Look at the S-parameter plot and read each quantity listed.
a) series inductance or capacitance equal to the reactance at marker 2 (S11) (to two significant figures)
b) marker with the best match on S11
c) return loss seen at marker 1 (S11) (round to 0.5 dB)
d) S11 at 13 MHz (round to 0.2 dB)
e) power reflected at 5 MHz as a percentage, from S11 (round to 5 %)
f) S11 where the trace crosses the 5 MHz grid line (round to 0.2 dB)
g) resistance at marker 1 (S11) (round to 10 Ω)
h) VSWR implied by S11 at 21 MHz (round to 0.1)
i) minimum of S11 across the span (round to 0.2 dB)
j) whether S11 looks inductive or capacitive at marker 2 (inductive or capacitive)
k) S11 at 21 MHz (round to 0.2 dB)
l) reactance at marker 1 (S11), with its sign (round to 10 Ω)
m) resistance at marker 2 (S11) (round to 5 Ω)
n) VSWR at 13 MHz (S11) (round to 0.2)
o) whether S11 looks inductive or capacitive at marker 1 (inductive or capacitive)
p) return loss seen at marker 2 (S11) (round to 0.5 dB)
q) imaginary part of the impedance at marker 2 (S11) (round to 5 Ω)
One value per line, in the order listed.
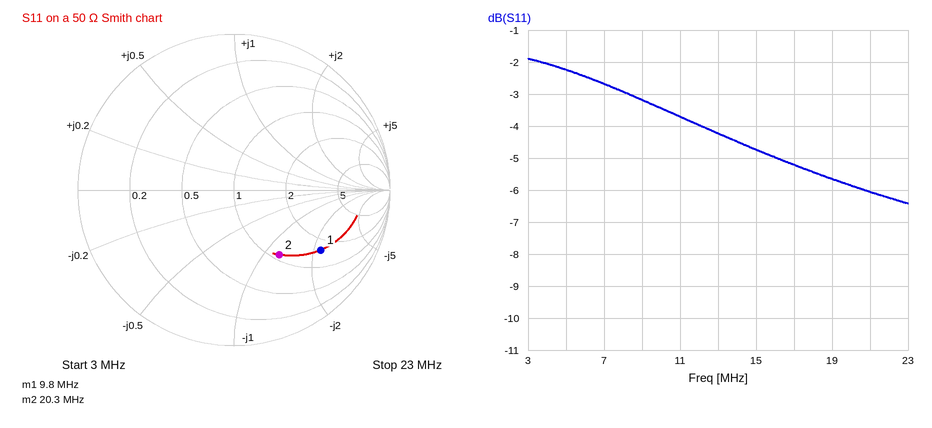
130 pF
marker 2
3.5 dB
-4.2 dB
60 %
-2.2 dB
80 Ω
3.0
-6.4 dB
capacitive
-6.0 dB
-110 Ω
55 Ω
4.2
capacitive
6.0 dB
-60 Ω
